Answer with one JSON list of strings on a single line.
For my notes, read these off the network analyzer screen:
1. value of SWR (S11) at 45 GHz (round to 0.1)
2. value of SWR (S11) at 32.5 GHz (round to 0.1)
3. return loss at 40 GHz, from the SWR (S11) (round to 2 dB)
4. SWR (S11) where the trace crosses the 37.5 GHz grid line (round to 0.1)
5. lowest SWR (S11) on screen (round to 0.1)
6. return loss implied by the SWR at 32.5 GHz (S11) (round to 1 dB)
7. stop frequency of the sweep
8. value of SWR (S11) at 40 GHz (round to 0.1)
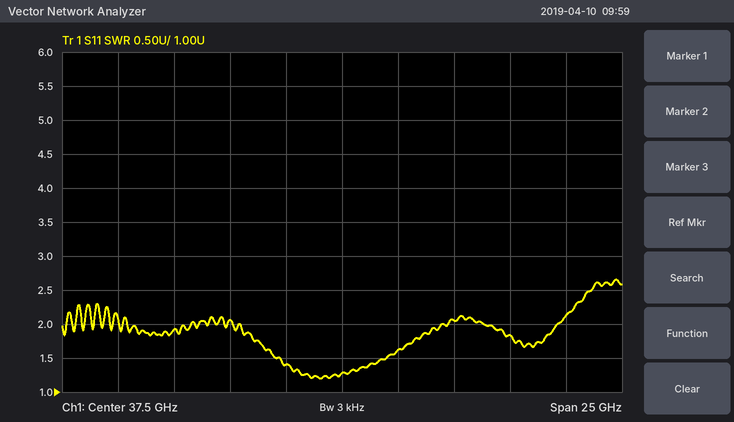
["1.8", "2.1", "12 dB", "1.3", "1.2", "9 dB", "50 GHz", "1.6"]
